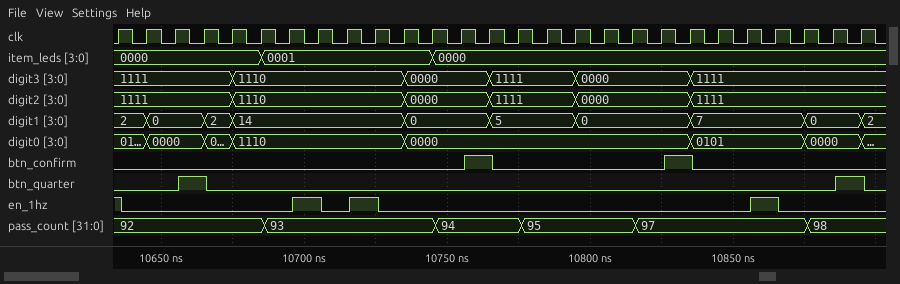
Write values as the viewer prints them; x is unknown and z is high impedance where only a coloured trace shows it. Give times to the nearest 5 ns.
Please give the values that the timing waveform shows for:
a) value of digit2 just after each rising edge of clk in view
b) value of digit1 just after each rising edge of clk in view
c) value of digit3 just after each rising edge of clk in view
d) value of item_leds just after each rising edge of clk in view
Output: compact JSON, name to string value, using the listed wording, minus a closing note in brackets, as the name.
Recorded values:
{"value of digit2 just after each rising edge of clk in view": "1111, 1111, 1111, 1111, 1110, 1110, 1110, 1110, 1110, 1110, 0000, 0000, 0000, 1111, 1111, 1111, 0000, 0000, 0000, 0000, 1111, 1111, 1111, 1111, 1111, 1111, 1111", "value of digit1 just after each rising edge of clk in view": "2, 0, 0, 2, 14, 14, 14, 14, 14, 14, 0, 0, 0, 5, 5, 5, 0, 0, 0, 0, 7, 7, 7, 7, 0, 0, 2", "value of digit3 just after each rising edge of clk in view": "1111, 1111, 1111, 1111, 1110, 1110, 1110, 1110, 1110, 1110, 0000, 0000, 0000, 1111, 1111, 1111, 0000, 0000, 0000, 0000, 1111, 1111, 1111, 1111, 1111, 1111, 1111", "value of item_leds just after each rising edge of clk in view": "0000, 0000, 0000, 0000, 0000, 0001, 0001, 0001, 0001, 0001, 0001, 0000, 0000, 0000, 0000, 0000, 0000, 0000, 0000, 0000, 0000, 0000, 0000, 0000, 0000, 0000, 0000"}
